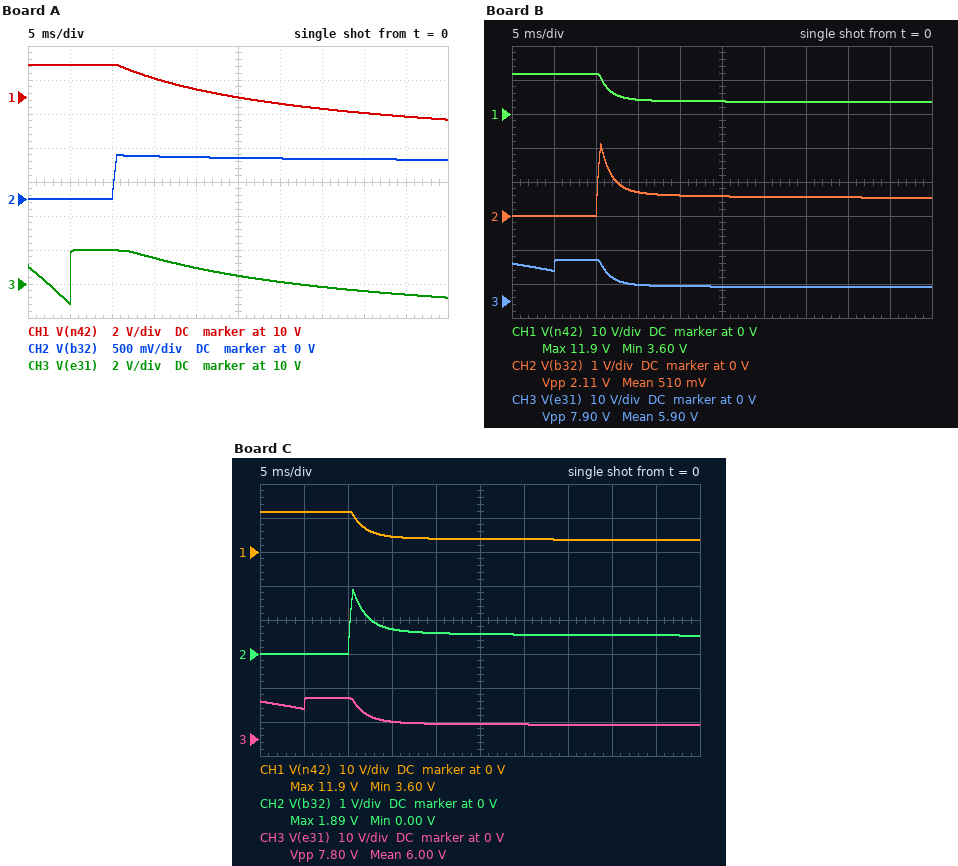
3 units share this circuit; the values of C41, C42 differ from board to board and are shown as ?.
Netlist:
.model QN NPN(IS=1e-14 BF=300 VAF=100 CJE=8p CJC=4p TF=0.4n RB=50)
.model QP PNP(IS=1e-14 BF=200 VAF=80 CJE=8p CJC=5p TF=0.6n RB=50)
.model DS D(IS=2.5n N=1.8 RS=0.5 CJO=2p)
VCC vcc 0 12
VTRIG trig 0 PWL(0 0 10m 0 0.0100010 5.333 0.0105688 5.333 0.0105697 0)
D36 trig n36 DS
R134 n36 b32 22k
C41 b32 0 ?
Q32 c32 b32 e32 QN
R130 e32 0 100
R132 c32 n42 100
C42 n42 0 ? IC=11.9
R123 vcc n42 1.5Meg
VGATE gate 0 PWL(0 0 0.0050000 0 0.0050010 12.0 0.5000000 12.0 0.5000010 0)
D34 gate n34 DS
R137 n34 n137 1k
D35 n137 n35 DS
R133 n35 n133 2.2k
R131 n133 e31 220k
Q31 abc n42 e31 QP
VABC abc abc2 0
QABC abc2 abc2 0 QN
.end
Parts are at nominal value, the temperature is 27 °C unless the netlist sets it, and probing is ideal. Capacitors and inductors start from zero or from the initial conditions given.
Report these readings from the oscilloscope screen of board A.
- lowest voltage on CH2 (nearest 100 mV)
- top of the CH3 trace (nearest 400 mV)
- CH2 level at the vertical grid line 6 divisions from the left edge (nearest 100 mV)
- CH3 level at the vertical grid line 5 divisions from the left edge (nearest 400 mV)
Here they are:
0 V
12.0 V
600 mV
10.4 V
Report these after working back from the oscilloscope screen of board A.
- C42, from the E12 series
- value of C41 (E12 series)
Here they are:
1.2 µF
180 nF
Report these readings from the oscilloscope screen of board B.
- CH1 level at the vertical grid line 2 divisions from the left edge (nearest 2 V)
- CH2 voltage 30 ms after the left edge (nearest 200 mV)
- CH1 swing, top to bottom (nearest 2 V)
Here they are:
12 V
600 mV
8 V
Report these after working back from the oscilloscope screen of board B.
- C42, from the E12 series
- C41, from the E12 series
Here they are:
2.7 µF
39 nF
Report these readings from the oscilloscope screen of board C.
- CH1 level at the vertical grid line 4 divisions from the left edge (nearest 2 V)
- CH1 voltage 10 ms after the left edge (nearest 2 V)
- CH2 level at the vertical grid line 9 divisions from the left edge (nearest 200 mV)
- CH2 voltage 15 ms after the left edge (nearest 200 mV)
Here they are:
4 V
12 V
600 mV
800 mV
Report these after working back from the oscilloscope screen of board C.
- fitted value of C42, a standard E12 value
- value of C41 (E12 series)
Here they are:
2.7 µF
47 nF
